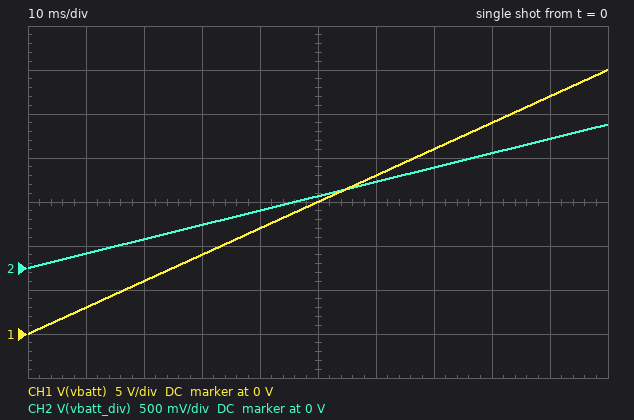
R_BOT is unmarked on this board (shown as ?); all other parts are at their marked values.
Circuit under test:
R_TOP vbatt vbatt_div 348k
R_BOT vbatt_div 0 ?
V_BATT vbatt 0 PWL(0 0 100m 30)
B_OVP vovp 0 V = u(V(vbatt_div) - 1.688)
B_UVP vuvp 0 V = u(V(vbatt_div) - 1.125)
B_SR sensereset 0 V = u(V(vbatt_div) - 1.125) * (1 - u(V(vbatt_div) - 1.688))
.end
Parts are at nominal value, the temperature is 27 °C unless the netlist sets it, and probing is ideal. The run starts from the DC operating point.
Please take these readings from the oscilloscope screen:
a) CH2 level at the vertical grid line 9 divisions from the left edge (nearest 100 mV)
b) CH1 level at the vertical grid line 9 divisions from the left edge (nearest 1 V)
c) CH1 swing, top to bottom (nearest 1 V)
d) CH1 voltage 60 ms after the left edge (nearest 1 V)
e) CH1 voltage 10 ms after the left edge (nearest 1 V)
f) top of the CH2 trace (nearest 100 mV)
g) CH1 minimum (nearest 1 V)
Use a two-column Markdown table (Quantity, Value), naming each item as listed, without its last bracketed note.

| Quantity | Value |
|---|---|
| CH2 level at the vertical grid line 9 divisions from the left edge | 1.5 V |
| CH1 level at the vertical grid line 9 divisions from the left edge | 27 V |
| CH1 swing, top to bottom | 30 V |
| CH1 voltage 60 ms after the left edge | 18 V |
| CH1 voltage 10 ms after the left edge | 3 V |
| top of the CH2 trace | 1.6 V |
| CH1 minimum | 0 V |
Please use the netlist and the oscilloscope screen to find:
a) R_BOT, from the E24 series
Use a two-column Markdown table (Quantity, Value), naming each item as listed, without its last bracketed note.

| Quantity | Value |
|---|---|
| R_BOT, from the E24 series | 20 kΩ |
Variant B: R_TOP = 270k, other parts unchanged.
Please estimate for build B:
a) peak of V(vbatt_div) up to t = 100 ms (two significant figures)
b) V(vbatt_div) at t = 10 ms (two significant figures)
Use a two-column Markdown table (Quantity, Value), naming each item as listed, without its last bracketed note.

| Quantity | Value |
|---|---|
| peak of V(vbatt_div) up to t = 100 ms | 2.1 V |
| V(vbatt_div) at t = 10 ms | 210 mV |
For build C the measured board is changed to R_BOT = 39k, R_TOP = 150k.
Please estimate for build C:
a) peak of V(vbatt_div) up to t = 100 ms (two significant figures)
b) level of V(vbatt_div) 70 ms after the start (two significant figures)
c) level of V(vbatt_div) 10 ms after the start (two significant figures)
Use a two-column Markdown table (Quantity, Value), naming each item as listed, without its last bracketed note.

| Quantity | Value |
|---|---|
| peak of V(vbatt_div) up to t = 100 ms | 6.2 V |
| level of V(vbatt_div) 70 ms after the start | 4.3 V |
| level of V(vbatt_div) 10 ms after the start | 620 mV |
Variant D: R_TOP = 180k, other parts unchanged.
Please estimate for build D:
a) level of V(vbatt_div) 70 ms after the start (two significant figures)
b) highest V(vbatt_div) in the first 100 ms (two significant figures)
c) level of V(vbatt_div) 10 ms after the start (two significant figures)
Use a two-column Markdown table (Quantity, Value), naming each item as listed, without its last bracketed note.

| Quantity | Value |
|---|---|
| level of V(vbatt_div) 70 ms after the start | 2.1 V |
| highest V(vbatt_div) in the first 100 ms | 3.0 V |
| level of V(vbatt_div) 10 ms after the start | 300 mV |
